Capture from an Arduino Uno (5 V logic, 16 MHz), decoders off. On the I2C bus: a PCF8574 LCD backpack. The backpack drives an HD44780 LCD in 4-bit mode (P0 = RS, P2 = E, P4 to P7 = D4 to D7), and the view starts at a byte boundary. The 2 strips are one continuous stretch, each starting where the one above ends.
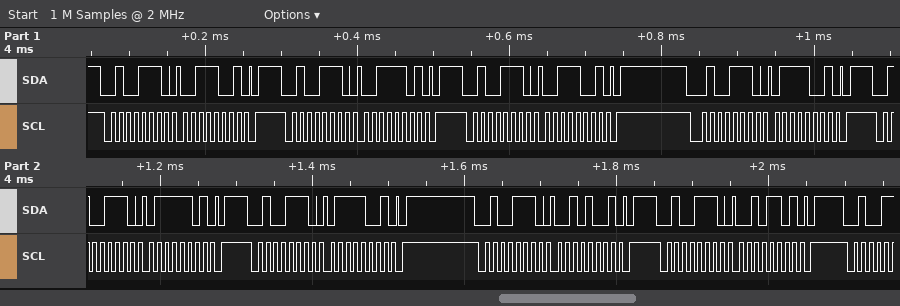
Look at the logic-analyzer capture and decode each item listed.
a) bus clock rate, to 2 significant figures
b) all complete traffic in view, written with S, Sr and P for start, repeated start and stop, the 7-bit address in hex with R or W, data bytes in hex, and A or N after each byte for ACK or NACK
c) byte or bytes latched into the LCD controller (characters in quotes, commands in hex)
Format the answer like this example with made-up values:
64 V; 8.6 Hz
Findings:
100 kHz; S 27W A 39 A P S 27W A 3D A P S 27W A 39 A P S 27W A 79 A P S 27W A 7D A P S 27W A 79 A P S 27W A 29 A P S 27W A 2D A P; '7'
